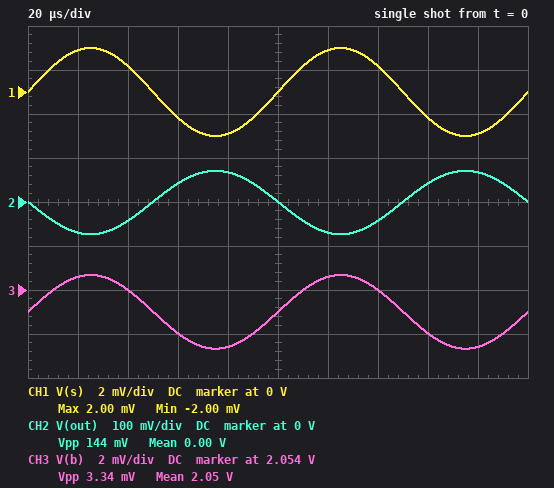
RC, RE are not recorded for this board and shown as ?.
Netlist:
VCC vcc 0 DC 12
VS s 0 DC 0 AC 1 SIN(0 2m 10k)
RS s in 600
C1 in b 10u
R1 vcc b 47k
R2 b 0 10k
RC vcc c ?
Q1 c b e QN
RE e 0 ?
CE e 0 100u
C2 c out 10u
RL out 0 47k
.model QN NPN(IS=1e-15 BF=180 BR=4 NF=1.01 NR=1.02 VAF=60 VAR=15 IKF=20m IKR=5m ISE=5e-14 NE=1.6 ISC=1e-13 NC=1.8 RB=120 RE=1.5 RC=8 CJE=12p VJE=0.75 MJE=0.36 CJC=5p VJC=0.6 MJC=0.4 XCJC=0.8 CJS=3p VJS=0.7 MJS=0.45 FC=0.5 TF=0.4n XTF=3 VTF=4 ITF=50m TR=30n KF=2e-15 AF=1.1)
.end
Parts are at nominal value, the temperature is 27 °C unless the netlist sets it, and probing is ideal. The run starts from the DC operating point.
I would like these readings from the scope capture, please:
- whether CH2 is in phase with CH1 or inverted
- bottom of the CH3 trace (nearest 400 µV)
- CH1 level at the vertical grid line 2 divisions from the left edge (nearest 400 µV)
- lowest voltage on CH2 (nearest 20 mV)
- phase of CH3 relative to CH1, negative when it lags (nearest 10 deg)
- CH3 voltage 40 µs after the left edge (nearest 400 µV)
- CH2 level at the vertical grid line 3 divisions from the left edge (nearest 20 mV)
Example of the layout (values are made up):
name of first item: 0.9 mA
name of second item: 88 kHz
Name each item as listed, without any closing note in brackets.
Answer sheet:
whether CH2 is in phase with CH1 or inverted: inverted
bottom of the CH3 trace: 2.0512 V
CH1 level at the vertical grid line 2 divisions from the left edge: 1.2 mV
lowest voltage on CH2: -80 mV
phase of CH3 relative to CH1, negative when it lags: 0 deg
CH3 voltage 40 µs after the left edge: 2.0540 V
CH2 level at the vertical grid line 3 divisions from the left edge: 40 mV
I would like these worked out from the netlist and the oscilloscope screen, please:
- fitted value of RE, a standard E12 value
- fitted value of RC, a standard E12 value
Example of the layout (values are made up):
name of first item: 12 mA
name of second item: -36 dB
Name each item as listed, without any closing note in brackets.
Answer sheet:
fitted value of RE, a standard E12 value: 1.5 kΩ
fitted value of RC, a standard E12 value: 1.5 kΩ
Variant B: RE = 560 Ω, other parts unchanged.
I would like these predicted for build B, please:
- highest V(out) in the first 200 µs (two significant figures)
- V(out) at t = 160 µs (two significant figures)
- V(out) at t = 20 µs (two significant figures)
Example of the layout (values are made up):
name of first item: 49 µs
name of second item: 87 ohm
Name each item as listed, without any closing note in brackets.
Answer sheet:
highest V(out) in the first 200 µs: 130 mV
V(out) at t = 160 µs: 78 mV
V(out) at t = 20 µs: -130 mV
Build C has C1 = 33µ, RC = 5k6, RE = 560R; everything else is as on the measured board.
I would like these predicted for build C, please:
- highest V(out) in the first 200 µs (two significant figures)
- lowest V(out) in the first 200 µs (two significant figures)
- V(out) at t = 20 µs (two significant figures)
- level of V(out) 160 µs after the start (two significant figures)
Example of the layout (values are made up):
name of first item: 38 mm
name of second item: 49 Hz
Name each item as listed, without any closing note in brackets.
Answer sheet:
highest V(out) in the first 200 µs: 4.3 mV
lowest V(out) in the first 200 µs: -3.7 mV
V(out) at t = 20 µs: -3.5 mV
level of V(out) 160 µs after the start: 2.4 mV
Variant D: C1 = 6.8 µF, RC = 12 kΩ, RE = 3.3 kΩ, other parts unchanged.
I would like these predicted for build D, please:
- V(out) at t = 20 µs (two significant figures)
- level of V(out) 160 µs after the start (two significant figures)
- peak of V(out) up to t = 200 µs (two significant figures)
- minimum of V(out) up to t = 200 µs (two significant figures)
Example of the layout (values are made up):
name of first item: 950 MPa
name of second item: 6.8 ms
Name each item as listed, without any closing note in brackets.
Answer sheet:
V(out) at t = 20 µs: -230 mV
level of V(out) 160 µs after the start: 140 mV
peak of V(out) up to t = 200 µs: 230 mV
minimum of V(out) up to t = 200 µs: -240 mV
